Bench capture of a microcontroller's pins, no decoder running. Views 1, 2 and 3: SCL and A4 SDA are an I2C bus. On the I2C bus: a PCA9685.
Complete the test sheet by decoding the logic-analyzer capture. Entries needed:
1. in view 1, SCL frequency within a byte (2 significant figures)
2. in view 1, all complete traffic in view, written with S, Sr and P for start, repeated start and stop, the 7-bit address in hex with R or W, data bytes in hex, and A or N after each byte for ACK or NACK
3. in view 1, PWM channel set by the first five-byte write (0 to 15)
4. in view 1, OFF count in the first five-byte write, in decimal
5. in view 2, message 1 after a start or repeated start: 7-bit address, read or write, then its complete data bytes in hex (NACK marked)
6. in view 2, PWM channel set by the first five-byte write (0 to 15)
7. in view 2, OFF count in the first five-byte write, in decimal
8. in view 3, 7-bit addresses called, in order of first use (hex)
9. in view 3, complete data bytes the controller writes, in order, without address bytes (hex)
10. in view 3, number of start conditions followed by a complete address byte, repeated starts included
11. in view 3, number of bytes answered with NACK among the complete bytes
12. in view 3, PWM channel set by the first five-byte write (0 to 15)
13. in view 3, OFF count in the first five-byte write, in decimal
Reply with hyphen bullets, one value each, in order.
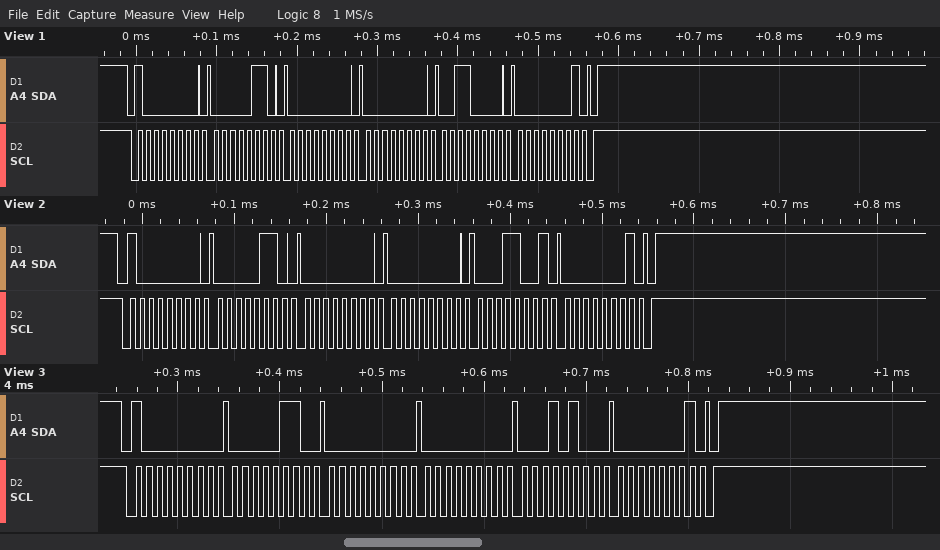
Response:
- 100 kHz
- S 40W A 06 A 00 A 00 A 30 A 01 A P
- 0
- 304
- 0x40 write: 06 00 00 19 01
- 0
- 281
- 0x40
- 06 00 00 14 01
- 1
- 0
- 0
- 276
